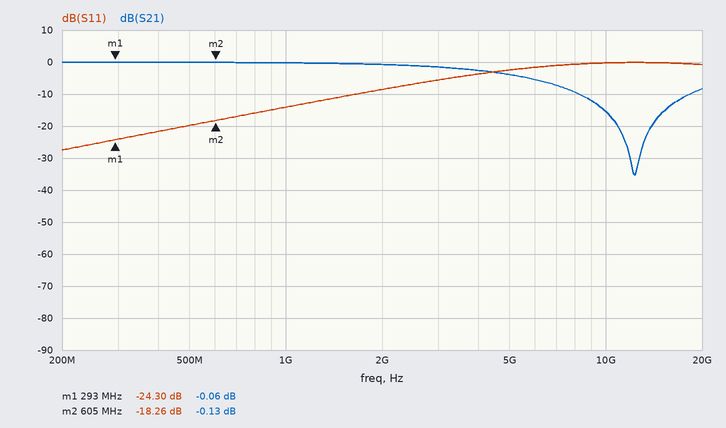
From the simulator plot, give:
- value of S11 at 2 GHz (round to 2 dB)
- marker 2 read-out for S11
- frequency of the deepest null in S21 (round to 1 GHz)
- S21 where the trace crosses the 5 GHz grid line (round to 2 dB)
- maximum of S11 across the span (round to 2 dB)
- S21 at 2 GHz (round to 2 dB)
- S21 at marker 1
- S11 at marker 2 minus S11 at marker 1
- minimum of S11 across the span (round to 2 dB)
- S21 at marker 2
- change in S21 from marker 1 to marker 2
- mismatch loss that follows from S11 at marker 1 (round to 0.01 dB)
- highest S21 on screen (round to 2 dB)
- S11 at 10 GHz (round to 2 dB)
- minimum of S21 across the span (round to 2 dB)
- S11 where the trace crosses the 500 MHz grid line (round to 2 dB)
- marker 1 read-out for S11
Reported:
-8 dB
-18.26 dB
12 GHz
-4 dB
0 dB
0 dB
-0.06 dB
6.04 dB
-28 dB
-0.13 dB
-0.07 dB
0.02 dB
0 dB
0 dB
-36 dB
-20 dB
-24.30 dB
